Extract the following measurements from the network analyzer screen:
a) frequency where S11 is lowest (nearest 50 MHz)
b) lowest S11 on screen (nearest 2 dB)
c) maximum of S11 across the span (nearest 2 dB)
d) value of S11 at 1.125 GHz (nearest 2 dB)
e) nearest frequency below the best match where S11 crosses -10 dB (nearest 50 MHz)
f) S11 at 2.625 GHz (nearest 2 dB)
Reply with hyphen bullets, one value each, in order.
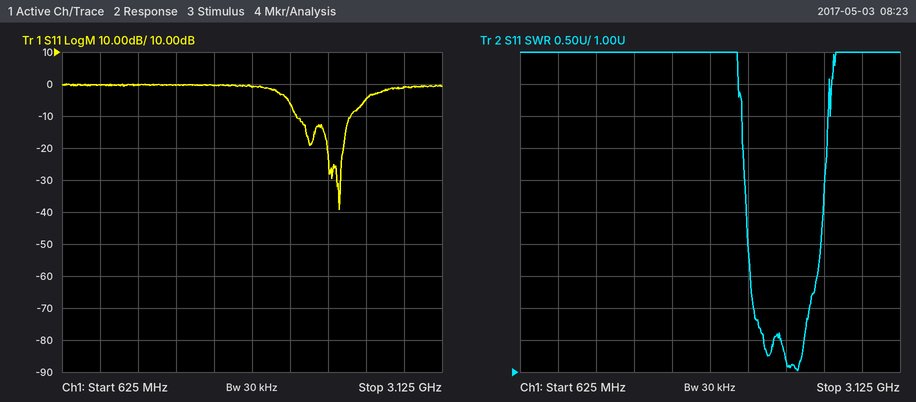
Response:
- 2.45 GHz
- -40 dB
- 0 dB
- 0 dB
- 2.15 GHz
- -4 dB
